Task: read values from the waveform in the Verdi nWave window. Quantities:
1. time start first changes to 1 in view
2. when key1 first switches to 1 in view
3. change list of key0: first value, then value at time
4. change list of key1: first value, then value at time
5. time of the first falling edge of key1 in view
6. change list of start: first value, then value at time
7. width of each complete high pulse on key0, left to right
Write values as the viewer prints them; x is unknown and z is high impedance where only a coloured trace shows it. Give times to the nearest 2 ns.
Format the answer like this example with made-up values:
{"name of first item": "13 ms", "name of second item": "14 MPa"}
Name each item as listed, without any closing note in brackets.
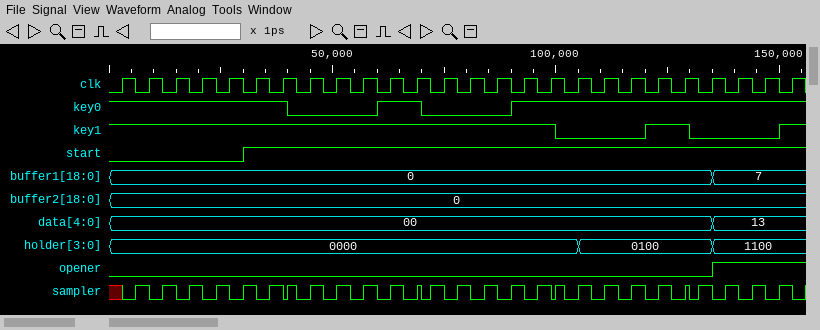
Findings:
{"time start first changes to 1 in view": "30 ns", "when key1 first switches to 1 in view": "120 ns", "change list of key0: first value, then value at time": "1, 0 at 40 ns, 1 at 60 ns, 0 at 70 ns, 1 at 90 ns", "change list of key1: first value, then value at time": "1, 0 at 100 ns, 1 at 120 ns, 0 at 130 ns, 1 at 150 ns", "time of the first falling edge of key1 in view": "100 ns", "change list of start: first value, then value at time": "0, 1 at 30 ns", "width of each complete high pulse on key0, left to right": "10 ns"}
